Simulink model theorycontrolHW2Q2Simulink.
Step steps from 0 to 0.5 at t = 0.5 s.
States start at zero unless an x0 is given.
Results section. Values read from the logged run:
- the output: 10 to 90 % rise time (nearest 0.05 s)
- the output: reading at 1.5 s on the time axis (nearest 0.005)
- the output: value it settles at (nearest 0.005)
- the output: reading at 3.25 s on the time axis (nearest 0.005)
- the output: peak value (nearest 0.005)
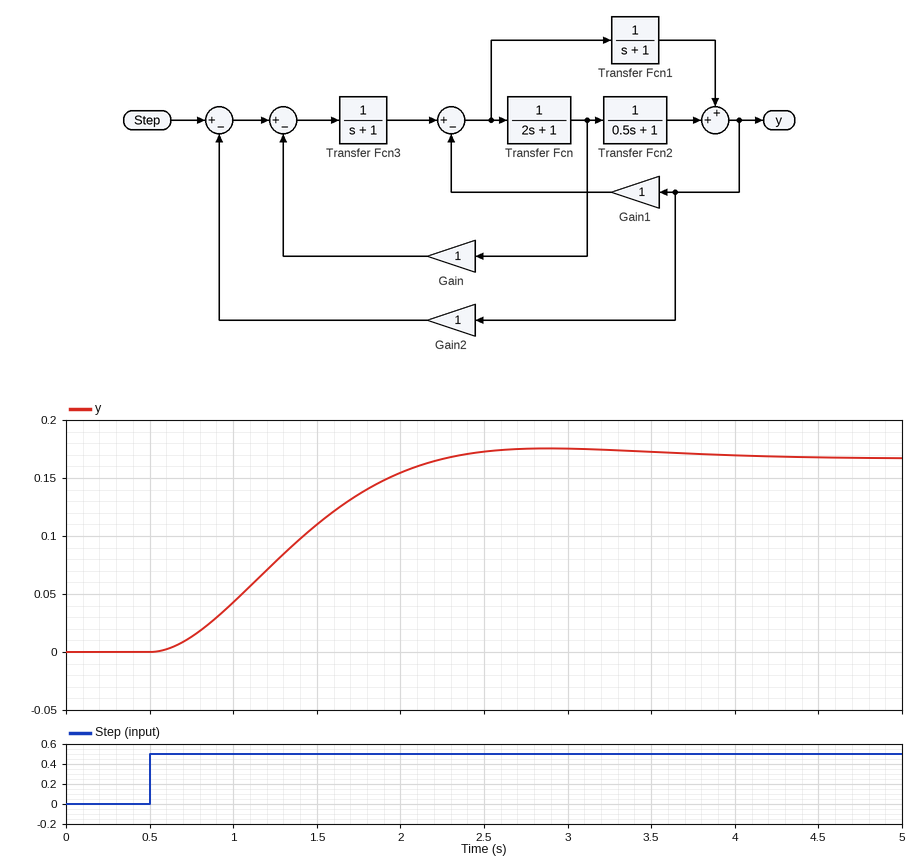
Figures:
1.15 s
0.110
0.165
0.175
0.175
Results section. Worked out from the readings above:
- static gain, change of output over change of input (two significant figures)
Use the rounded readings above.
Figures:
0.33
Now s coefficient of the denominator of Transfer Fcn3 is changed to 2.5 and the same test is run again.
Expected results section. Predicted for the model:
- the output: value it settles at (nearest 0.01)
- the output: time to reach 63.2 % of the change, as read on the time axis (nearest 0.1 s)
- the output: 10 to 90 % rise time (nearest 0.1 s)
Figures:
0.17
2.2 s
2.4 s
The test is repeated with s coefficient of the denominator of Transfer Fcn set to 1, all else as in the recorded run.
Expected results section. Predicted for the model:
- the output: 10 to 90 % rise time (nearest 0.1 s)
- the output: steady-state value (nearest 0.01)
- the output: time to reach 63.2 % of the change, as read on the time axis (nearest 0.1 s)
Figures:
1.0 s
0.17
1.4 s
